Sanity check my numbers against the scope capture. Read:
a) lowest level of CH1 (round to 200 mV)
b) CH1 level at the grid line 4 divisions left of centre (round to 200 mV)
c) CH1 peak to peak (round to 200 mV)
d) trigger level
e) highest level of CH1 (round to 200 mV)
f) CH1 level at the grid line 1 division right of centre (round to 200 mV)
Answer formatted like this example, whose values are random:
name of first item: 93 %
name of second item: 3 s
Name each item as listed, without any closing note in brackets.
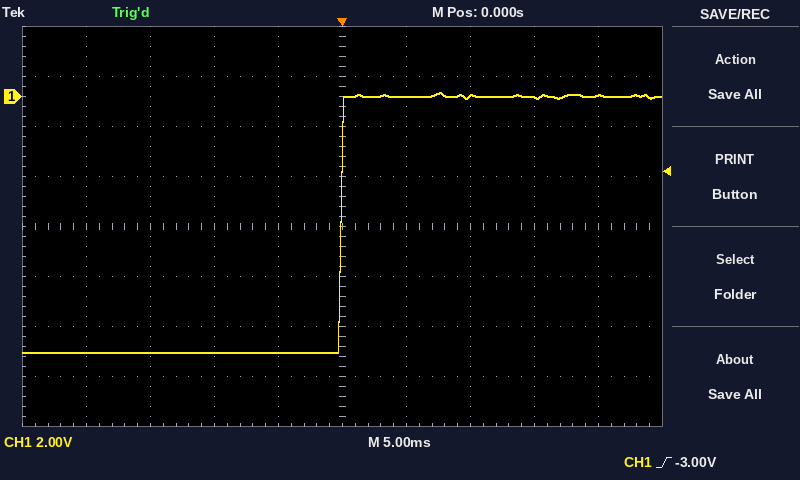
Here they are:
lowest level of CH1: -10.2 V
CH1 level at the grid line 4 divisions left of centre: -10.2 V
CH1 peak to peak: 10.4 V
trigger level: -3.00 V
highest level of CH1: 200 mV
CH1 level at the grid line 1 division right of centre: 0.0 V
